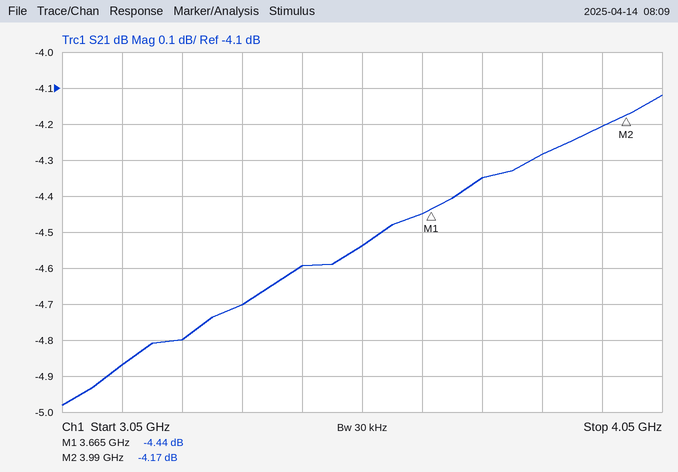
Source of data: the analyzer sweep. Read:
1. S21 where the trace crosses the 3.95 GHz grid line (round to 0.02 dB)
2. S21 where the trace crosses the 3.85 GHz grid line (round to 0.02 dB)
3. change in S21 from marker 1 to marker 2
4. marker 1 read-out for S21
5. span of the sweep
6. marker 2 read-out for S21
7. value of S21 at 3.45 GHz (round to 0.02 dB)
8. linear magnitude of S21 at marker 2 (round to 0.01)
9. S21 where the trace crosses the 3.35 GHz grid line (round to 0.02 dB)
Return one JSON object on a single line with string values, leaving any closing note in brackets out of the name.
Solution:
{"S21 where the trace crosses the 3.95 GHz grid line": "-4.20 dB", "S21 where the trace crosses the 3.85 GHz grid line": "-4.28 dB", "change in S21 from marker 1 to marker 2": "0.27 dB", "marker 1 read-out for S21": "-4.44 dB", "span of the sweep": "1 GHz", "marker 2 read-out for S21": "-4.17 dB", "value of S21 at 3.45 GHz": "-4.60 dB", "linear magnitude of S21 at marker 2": "0.62", "S21 where the trace crosses the 3.35 GHz grid line": "-4.70 dB"}
